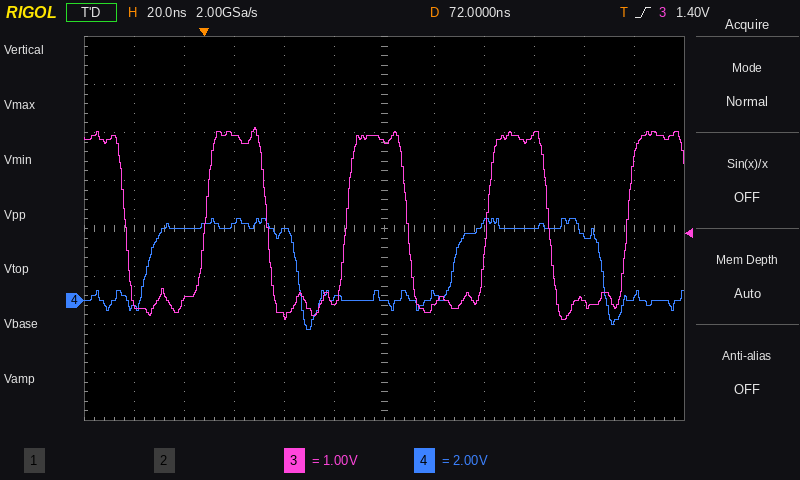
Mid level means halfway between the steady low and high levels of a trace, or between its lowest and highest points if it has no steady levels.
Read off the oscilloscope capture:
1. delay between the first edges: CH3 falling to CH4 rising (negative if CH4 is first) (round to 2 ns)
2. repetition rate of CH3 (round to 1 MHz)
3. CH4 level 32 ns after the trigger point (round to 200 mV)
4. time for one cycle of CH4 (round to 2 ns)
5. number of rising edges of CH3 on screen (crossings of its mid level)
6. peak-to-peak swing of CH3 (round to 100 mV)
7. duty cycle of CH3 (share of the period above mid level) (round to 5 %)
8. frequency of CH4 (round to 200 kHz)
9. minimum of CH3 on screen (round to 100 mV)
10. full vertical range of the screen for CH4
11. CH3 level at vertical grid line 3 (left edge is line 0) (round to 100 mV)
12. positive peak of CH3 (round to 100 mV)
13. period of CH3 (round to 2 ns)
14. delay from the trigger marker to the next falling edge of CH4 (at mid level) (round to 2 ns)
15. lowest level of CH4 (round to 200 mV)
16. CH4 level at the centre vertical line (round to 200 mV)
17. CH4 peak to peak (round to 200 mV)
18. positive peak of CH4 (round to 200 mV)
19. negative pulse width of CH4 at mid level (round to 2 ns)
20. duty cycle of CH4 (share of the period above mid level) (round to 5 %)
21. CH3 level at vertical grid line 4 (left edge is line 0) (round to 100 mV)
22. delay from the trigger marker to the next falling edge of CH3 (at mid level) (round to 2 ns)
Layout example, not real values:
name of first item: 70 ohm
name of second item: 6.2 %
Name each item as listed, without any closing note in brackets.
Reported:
delay between the first edges: CH3 falling to CH4 rising (negative if CH4 is first): +8 ns
repetition rate of CH3: 18 MHz
CH4 level 32 ns after the trigger point: 3.0 V
time for one cycle of CH4: 122 ns
number of rising edges of CH3 on screen: 4
peak-to-peak swing of CH3: 4.0 V
duty cycle of CH3 (share of the period above mid level): 45 %
frequency of CH4: 8.2 MHz
minimum of CH3 on screen: -400 mV
full vertical range of the screen for CH4: 16 V
CH3 level at vertical grid line 3 (left edge is line 0): 3.5 V
positive peak of CH3: 3.6 V
period of CH3: 56 ns
delay from the trigger marker to the next falling edge of CH4 (at mid level): 38 ns
lowest level of CH4: -1.2 V
CH4 level at the centre vertical line: 0.0 V
CH4 peak to peak: 4.6 V
positive peak of CH4: 3.4 V
negative pulse width of CH4 at mid level: 62 ns
duty cycle of CH4 (share of the period above mid level): 50 %
CH3 level at vertical grid line 4 (left edge is line 0): -300 mV
delay from the trigger marker to the next falling edge of CH3 (at mid level): 26 ns
